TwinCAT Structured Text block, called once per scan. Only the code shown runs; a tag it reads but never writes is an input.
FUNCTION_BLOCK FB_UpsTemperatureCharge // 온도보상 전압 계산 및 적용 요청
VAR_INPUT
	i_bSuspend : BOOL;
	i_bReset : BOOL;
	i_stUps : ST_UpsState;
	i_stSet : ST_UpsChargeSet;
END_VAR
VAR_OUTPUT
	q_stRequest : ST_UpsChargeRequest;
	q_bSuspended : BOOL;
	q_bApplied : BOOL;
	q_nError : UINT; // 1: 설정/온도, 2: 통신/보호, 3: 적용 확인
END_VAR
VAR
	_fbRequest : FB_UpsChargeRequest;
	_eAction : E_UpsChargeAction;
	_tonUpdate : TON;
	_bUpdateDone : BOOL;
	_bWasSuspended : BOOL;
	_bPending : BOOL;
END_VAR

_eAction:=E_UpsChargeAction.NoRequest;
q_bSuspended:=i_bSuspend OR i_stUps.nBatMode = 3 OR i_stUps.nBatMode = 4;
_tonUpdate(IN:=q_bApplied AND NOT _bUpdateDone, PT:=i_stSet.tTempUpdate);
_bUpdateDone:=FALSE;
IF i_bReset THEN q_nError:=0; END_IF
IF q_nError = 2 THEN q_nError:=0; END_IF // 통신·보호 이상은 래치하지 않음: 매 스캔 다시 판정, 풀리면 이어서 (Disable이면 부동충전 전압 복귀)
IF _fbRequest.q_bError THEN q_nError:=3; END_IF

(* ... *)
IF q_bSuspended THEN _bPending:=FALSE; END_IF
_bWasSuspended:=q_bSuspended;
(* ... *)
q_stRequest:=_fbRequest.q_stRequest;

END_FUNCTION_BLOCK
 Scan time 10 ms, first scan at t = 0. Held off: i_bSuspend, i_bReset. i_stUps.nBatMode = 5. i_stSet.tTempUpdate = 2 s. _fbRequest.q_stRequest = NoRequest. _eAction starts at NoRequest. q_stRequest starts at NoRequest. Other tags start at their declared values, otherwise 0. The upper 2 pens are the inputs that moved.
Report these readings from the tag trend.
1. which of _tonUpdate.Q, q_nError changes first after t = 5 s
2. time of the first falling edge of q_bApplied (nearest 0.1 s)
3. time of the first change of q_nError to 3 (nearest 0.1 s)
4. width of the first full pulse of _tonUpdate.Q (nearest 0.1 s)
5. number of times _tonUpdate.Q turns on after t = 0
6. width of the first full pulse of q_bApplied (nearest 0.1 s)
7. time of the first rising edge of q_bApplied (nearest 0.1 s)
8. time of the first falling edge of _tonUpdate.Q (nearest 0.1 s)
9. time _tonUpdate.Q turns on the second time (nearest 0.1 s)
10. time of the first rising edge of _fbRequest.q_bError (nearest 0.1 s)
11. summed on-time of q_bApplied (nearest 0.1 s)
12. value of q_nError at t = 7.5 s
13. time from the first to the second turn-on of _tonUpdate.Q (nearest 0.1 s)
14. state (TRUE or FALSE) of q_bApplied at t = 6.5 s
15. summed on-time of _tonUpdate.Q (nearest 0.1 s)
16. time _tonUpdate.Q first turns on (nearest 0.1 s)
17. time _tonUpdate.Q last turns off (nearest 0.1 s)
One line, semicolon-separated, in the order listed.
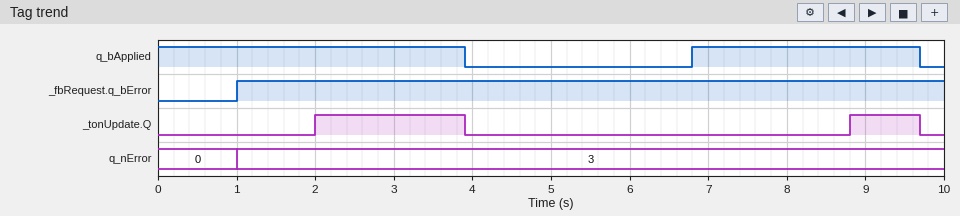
_tonUpdate.Q; 3.9 s; 1.0 s; 1.9 s; 2; 2.9 s; 6.8 s; 3.9 s; 8.8 s; 1.0 s; 6.8 s; 3; 6.8 s; FALSE; 2.8 s; 2.0 s; 9.7 s
